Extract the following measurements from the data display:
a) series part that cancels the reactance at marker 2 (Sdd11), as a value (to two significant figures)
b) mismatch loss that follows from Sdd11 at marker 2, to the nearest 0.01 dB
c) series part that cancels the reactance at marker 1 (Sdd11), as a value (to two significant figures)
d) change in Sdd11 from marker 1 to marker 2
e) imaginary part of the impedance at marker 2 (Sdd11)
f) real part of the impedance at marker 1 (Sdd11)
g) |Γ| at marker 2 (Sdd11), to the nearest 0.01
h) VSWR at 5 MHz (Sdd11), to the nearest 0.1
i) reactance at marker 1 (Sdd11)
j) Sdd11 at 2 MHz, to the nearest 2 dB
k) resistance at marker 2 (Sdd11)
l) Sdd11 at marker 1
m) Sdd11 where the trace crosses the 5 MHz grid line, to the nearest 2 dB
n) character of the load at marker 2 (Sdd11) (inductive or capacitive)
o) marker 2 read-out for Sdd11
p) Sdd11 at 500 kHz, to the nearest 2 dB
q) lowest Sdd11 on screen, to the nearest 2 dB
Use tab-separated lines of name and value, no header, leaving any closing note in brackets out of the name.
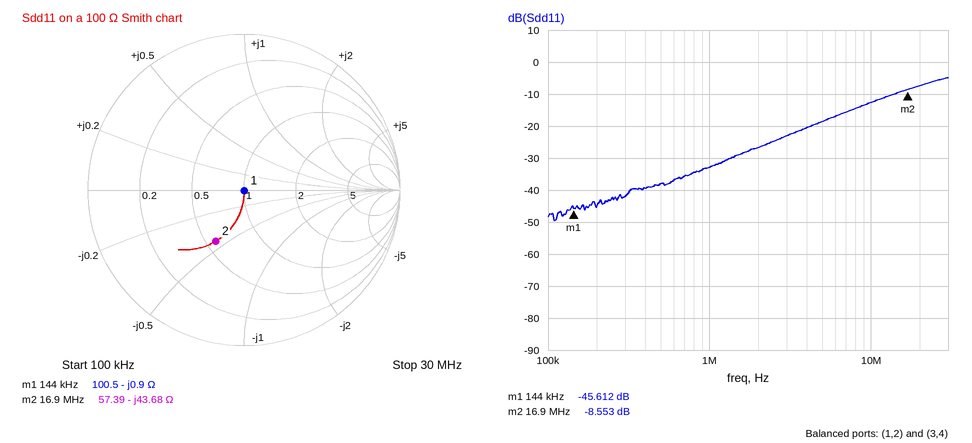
series part that cancels the reactance at marker 2 (Sdd11), as a value	410 nH
mismatch loss that follows from Sdd11 at marker 2, to the nearest 0.01 dB	0.65 dB
series part that cancels the reactance at marker 1 (Sdd11), as a value	1.0 µH
change in Sdd11 from marker 1 to marker 2	37.059 dB
imaginary part of the impedance at marker 2	-43.68 Ω
real part of the impedance at marker 1	100.5 Ω
|Γ| at marker 2 (Sdd11), to the nearest 0.01	0.37
VSWR at 5 MHz (Sdd11), to the nearest 0.1	1.3
reactance at marker 1	-0.9 Ω
Sdd11 at 2 MHz, to the nearest 2 dB	-26 dB
resistance at marker 2	57.39 Ω
Sdd11 at marker 1	-45.612 dB
Sdd11 where the trace crosses the 5 MHz grid line, to the nearest 2 dB	-18 dB
character of the load at marker 2 (Sdd11)	capacitive
marker 2 read-out for Sdd11	-8.553 dB
Sdd11 at 500 kHz, to the nearest 2 dB	-38 dB
lowest Sdd11 on screen, to the nearest 2 dB	-50 dB
